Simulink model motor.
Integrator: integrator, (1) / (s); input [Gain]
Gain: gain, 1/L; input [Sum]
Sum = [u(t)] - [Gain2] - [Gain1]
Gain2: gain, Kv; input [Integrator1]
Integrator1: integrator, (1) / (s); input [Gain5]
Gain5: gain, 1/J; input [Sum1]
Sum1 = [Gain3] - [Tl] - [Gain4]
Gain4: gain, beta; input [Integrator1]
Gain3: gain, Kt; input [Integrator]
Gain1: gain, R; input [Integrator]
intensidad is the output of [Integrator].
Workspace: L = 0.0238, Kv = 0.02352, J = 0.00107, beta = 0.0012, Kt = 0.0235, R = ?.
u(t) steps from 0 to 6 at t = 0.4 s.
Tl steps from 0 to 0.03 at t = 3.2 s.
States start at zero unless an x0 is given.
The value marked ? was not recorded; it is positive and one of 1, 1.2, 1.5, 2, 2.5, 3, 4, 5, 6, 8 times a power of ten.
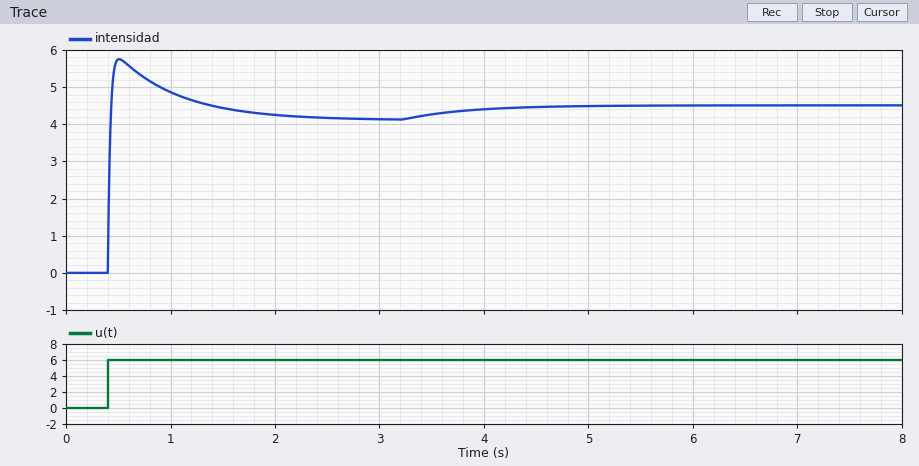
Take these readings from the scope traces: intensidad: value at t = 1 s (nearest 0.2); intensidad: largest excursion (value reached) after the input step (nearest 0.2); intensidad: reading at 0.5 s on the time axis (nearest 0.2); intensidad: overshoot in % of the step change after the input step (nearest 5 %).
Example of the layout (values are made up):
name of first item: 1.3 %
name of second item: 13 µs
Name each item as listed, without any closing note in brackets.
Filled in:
intensidad: value at t = 1 s: 4.8
intensidad: largest excursion (value reached) after the input step: 5.8
intensidad: reading at 0.5 s on the time axis: 5.8
intensidad: overshoot in % of the step change after the input step: 40 %
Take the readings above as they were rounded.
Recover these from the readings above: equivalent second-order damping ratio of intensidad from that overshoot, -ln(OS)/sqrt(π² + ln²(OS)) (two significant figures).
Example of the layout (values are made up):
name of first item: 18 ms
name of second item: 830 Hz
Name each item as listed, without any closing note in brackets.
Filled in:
equivalent second-order damping ratio of intensidad from that overshoot, -ln(OS)/sqrt(π² + ln²(OS)): 0.28
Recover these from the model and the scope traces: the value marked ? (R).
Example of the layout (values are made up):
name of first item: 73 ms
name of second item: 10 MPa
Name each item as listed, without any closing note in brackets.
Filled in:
the value marked ?: 1
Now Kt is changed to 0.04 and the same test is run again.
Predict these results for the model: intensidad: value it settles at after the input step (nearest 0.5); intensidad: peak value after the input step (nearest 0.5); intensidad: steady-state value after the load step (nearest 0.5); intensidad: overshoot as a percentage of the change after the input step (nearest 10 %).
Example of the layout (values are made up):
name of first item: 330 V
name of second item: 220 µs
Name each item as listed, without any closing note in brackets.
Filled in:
intensidad: value it settles at after the input step: 3.5
intensidad: peak value after the input step: 5.5
intensidad: steady-state value after the load step: 3.5
intensidad: overshoot as a percentage of the change after the input step: 70 %
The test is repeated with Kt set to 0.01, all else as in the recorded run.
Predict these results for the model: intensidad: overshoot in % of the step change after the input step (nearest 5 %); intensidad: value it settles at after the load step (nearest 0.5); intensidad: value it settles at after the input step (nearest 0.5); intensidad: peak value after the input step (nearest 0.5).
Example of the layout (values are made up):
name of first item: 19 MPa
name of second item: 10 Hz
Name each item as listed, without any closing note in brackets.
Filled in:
intensidad: overshoot in % of the step change after the input step: 15 %
intensidad: value it settles at after the load step: 5.5
intensidad: value it settles at after the input step: 5.0
intensidad: peak value after the input step: 6.0
